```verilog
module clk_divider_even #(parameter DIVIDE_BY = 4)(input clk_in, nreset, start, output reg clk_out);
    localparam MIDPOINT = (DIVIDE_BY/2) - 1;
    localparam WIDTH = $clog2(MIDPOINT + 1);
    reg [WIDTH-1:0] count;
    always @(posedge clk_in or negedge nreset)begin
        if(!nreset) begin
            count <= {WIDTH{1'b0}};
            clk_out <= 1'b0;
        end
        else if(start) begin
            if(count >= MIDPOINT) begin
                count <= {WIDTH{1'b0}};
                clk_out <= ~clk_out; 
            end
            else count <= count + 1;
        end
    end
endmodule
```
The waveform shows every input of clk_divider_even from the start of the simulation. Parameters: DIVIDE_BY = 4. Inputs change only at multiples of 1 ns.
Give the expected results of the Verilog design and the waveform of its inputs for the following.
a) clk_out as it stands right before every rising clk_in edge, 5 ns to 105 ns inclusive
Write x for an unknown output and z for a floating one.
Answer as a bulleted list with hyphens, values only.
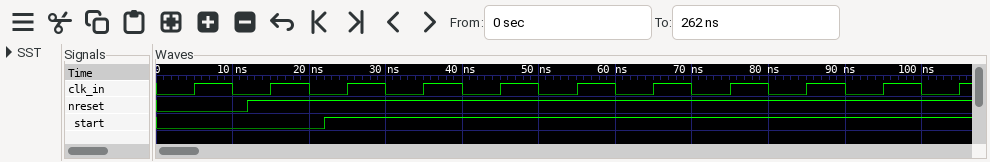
- 0 0 0 0 1 1 0 0 1 1 0
